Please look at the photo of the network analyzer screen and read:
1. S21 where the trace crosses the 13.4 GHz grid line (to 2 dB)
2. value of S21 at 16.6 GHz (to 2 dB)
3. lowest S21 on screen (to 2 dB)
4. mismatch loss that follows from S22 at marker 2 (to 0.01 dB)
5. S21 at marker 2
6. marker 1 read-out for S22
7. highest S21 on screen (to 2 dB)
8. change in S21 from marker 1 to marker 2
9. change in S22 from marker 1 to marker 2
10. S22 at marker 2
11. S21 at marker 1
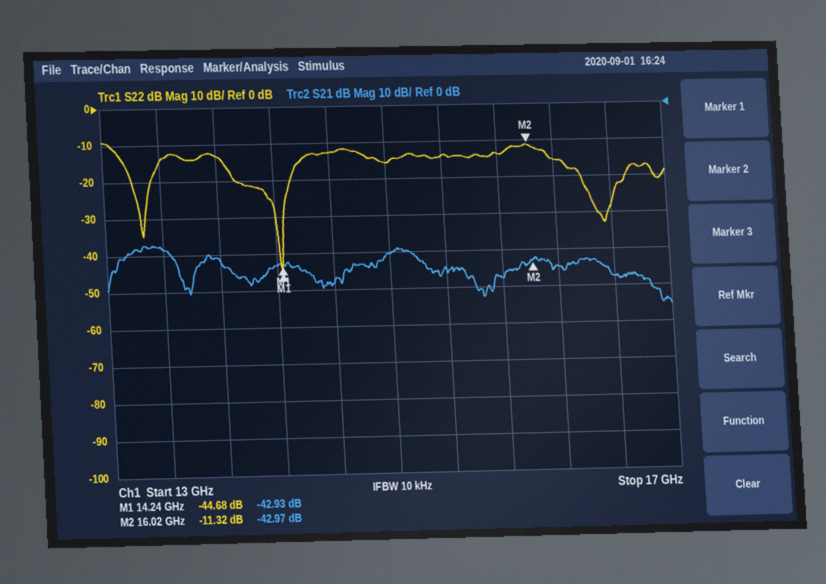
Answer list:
-38 dB
-48 dB
-56 dB
0.33 dB
-42.97 dB
-44.68 dB
-38 dB
-0.04 dB
33.36 dB
-11.32 dB
-42.93 dB
